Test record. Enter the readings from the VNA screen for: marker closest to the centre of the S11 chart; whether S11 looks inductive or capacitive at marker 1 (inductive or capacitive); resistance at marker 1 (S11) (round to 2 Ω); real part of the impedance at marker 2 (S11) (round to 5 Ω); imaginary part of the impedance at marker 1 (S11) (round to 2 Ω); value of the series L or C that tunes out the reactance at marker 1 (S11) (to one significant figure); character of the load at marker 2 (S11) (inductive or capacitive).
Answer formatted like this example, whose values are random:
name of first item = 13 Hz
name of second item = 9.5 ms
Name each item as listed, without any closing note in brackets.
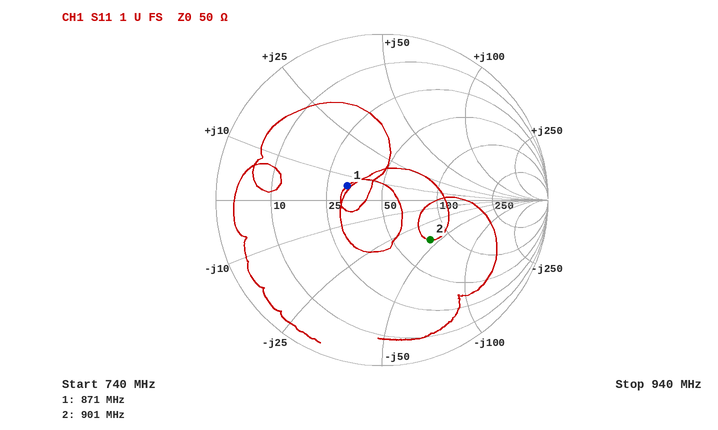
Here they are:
marker closest to the centre of the S11 chart = marker 1
whether S11 looks inductive or capacitive at marker 1 = inductive
resistance at marker 1 (S11) = 32 Ω
real part of the impedance at marker 2 (S11) = 75 Ω
imaginary part of the impedance at marker 1 (S11) = +6 Ω
value of the series L or C that tunes out the reactance at marker 1 (S11) = 30 pF
character of the load at marker 2 (S11) = capacitive
